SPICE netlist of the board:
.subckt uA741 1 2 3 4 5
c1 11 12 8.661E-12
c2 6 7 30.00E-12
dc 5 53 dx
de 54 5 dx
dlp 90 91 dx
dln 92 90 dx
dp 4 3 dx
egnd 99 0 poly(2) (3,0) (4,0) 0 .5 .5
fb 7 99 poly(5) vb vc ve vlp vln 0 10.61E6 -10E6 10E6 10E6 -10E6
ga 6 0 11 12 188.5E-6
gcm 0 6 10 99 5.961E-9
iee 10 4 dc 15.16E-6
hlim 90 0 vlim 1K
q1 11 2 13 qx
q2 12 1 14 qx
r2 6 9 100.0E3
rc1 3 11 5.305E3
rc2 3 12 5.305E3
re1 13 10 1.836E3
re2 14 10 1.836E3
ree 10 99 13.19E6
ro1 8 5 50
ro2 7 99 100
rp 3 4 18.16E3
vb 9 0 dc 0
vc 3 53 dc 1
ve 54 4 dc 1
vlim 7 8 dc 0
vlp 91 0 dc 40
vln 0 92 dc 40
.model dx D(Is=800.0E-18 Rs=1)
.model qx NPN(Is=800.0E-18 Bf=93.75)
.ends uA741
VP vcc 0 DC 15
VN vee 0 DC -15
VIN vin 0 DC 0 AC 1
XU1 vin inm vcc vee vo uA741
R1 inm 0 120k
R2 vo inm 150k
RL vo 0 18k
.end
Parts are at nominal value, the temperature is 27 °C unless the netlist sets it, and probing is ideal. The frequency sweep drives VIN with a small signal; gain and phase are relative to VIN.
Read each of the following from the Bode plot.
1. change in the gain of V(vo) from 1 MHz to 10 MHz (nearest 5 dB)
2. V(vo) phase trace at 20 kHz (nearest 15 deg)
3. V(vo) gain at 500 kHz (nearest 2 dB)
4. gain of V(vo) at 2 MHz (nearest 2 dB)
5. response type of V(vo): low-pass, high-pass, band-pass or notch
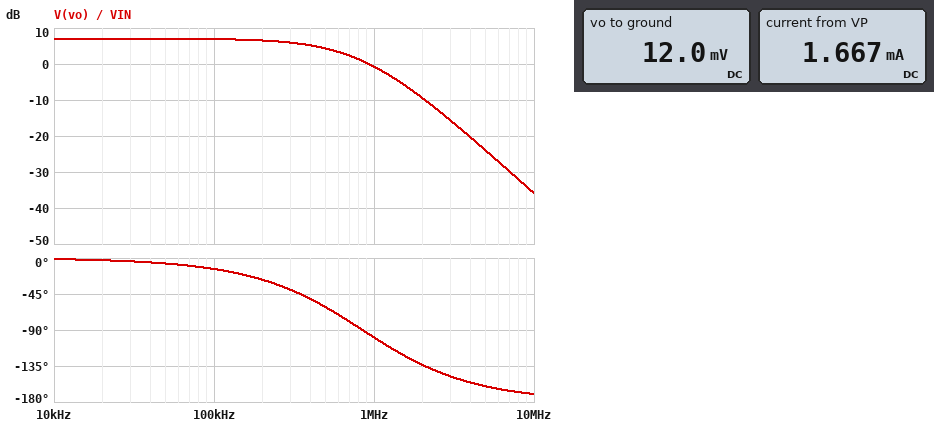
-35 dB
0 deg
4 dB
-10 dB
low-pass
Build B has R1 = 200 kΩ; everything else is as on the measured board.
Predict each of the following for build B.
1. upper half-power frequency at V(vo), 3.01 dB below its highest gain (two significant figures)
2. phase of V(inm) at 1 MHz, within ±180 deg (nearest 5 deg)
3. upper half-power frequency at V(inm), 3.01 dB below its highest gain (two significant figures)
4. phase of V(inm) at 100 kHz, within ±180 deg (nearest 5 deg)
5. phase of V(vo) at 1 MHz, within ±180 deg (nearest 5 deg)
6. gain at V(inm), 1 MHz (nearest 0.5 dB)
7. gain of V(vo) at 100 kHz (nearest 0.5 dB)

700 kHz
-85 deg
660 kHz
-10 deg
-95 deg
-6.5 dB
5.0 dB
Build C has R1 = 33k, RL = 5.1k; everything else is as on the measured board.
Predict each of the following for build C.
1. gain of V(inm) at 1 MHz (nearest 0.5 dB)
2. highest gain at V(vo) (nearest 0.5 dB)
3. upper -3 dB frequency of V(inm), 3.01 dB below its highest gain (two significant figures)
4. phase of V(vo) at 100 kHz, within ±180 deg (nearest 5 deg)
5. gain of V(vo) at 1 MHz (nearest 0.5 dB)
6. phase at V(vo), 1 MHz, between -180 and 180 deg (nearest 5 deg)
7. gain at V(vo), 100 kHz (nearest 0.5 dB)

-16.5 dB
15.0 dB
190 kHz
-30 deg
-1.0 dB
-110 deg
14.0 dB
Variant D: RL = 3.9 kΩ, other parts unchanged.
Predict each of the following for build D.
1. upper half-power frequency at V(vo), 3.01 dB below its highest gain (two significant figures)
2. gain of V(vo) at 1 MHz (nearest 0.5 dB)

520 kHz
-1.0 dB
